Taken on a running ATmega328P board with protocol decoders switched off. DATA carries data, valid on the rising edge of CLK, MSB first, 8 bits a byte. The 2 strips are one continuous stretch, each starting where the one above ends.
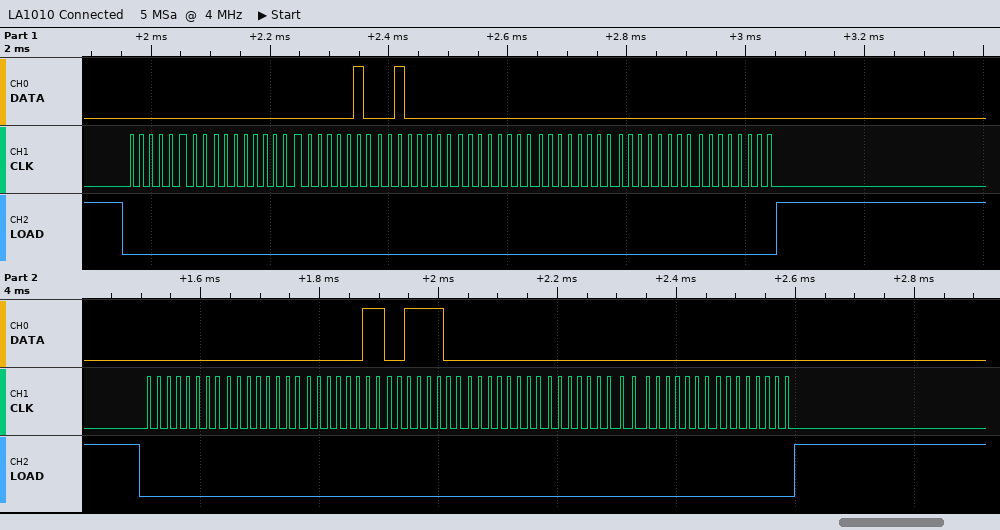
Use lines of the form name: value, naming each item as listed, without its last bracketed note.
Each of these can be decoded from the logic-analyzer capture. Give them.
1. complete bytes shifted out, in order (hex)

complete bytes shifted out, in order: 00 00 02 20 00 00 00 00 00 00 03 3C 00 00 00 00
